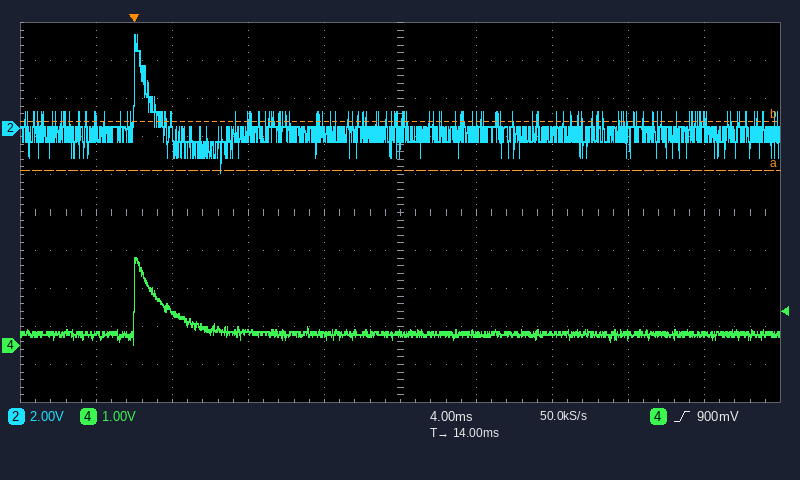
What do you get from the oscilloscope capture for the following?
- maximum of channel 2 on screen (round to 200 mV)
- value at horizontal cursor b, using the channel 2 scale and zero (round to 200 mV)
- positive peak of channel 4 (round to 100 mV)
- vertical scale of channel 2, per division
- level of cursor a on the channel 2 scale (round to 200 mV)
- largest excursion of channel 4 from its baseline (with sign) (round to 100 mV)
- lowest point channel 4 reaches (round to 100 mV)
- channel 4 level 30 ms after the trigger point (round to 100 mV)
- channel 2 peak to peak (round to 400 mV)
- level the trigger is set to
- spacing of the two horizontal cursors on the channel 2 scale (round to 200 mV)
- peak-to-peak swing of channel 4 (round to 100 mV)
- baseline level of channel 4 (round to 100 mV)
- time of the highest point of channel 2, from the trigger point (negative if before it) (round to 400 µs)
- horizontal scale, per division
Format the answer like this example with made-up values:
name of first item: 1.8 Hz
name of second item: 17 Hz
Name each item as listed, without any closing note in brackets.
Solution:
maximum of channel 2 on screen: 5.0 V
value at horizontal cursor b, using the channel 2 scale and zero: 400 mV
positive peak of channel 4: 2.3 V
vertical scale of channel 2, per division: 2 V
level of cursor a on the channel 2 scale: -2.2 V
largest excursion of channel 4 from its baseline (with sign): +2.0 V
lowest point channel 4 reaches: 0.0 V
channel 4 level 30 ms after the trigger point: 300 mV
channel 2 peak to peak: 7.2 V
level the trigger is set to: 900 mV
spacing of the two horizontal cursors on the channel 2 scale: 2.6 V
peak-to-peak swing of channel 4: 2.3 V
baseline level of channel 4: 300 mV
time of the highest point of channel 2, from the trigger point (negative if before it): 0.0 ms
horizontal scale, per division: 4 ms
